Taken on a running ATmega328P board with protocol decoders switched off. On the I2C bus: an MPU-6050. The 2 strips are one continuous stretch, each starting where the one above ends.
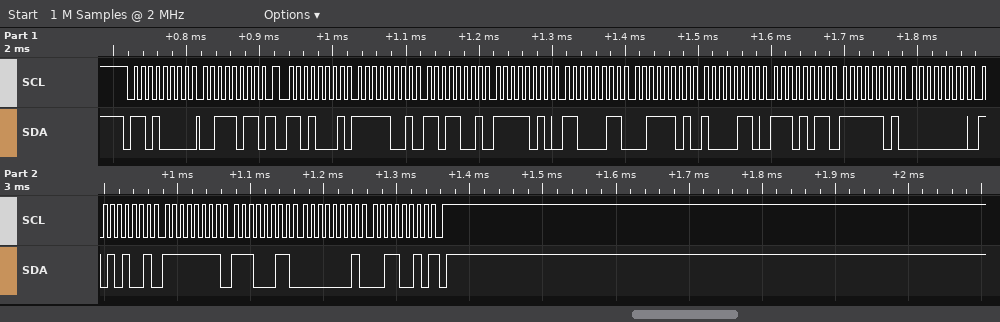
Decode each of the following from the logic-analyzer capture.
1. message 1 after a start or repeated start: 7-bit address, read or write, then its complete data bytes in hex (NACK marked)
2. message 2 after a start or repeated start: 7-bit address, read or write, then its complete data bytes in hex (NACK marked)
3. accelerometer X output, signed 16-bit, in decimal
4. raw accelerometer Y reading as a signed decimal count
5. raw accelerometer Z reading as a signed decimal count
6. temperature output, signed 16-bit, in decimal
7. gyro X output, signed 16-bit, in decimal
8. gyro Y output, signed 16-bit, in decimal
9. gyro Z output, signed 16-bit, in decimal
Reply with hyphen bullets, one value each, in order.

- 0x68 write: 3B
- 0x68 read: F9 D9 FA C3 3D 86 EB FD 00 A9 FF E3 01 32 NACK
- -1575
- -1341
- 15750
- -5123
- 169
- -29
- 306
